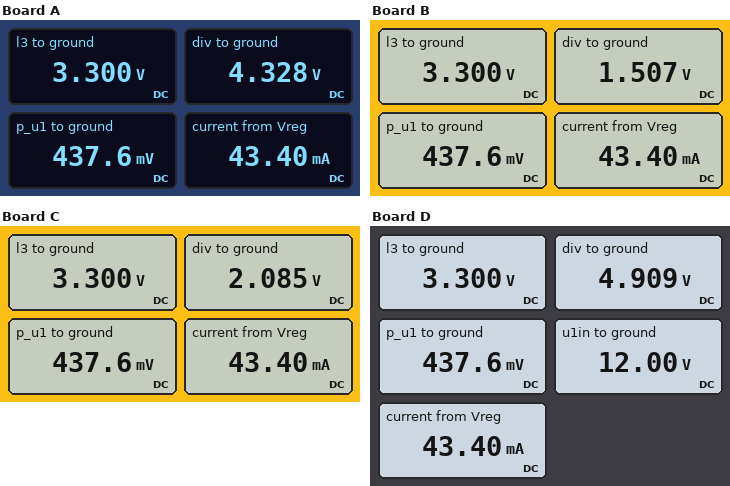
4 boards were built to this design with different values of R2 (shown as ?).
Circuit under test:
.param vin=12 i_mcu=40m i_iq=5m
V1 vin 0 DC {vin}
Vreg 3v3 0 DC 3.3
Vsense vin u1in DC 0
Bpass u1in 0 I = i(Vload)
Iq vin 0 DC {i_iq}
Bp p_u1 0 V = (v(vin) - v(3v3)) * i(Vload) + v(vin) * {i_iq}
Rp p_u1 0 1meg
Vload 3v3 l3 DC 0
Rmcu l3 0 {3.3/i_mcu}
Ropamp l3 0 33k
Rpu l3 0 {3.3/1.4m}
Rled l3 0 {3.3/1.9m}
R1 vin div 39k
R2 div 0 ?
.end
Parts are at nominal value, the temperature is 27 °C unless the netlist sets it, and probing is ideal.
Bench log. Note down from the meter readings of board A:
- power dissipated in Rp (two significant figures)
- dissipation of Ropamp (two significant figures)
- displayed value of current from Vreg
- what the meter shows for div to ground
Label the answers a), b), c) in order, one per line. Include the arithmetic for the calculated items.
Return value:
a) (437.6 mV)^2 / 1 MΩ = 190 nW
b) (3.3 V)^2 / 33 kΩ = 330 µW
c) 43.40 mA
d) 4.328 V
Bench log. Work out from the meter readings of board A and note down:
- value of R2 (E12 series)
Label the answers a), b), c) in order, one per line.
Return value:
a) 22 kΩ
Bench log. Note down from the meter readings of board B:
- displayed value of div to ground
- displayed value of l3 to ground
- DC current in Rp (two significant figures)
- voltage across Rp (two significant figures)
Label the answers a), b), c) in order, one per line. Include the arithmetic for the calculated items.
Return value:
a) 1.507 V
b) 3.300 V
c) (437.6 mV) / 1 MΩ = 440 nA
d) 437.6 mV = 440 mV
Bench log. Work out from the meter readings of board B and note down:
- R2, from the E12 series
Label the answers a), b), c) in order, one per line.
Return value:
a) 5.6 kΩ
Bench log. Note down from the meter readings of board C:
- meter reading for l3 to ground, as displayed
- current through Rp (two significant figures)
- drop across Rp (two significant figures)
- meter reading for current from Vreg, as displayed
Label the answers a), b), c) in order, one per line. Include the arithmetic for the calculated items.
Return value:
a) 3.300 V
b) (437.6 mV) / 1 MΩ = 440 nA
c) 437.6 mV = 440 mV
d) 43.40 mA
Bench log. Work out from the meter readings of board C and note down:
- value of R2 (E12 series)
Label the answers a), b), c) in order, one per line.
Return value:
a) 8.2 kΩ
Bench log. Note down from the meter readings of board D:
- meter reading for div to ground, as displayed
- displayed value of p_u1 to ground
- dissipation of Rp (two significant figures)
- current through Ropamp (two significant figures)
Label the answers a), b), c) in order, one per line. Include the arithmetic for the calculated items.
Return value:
a) 4.909 V
b) 437.6 mV
c) (437.6 mV)^2 / 1 MΩ = 190 nW
d) (3.3 V) / 33 kΩ = 100 µA
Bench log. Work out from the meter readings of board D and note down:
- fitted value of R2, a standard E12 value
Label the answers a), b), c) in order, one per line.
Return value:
a) 27 kΩ
